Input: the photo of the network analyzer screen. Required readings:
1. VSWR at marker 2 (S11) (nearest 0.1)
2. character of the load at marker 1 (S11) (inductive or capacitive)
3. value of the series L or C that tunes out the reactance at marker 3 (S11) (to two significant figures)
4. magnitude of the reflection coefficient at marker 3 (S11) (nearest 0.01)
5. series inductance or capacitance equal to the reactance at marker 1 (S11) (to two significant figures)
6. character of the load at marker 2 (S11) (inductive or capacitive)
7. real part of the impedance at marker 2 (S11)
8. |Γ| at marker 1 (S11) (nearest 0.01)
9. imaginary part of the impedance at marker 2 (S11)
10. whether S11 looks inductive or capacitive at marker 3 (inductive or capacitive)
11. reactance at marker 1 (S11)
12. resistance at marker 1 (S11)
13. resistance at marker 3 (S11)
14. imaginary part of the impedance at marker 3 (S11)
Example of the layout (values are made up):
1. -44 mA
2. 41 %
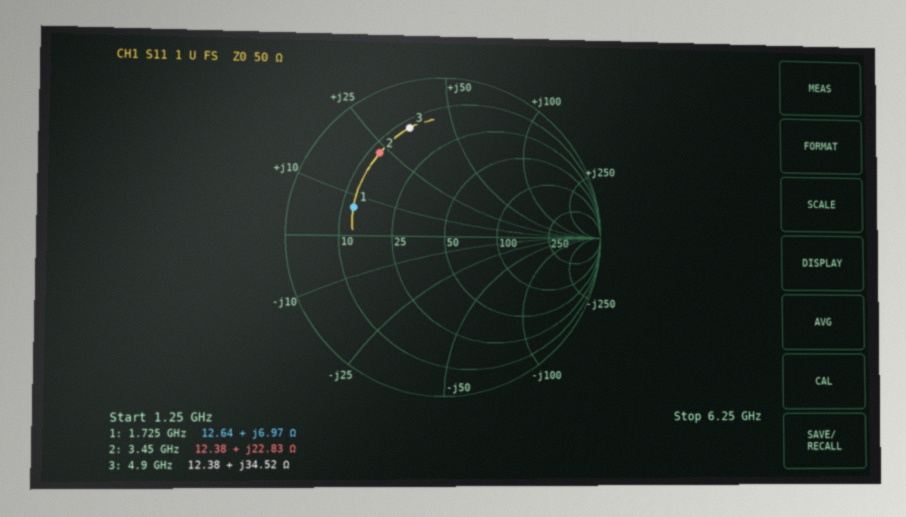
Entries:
1. 4.9
2. inductive
3. 940 fF
4. 0.72
5. 640 pH
6. inductive
7. 12.38 Ω
8. 0.60
9. +22.83 Ω
10. inductive
11. +6.97 Ω
12. 12.64 Ω
13. 12.38 Ω
14. +34.52 Ω
